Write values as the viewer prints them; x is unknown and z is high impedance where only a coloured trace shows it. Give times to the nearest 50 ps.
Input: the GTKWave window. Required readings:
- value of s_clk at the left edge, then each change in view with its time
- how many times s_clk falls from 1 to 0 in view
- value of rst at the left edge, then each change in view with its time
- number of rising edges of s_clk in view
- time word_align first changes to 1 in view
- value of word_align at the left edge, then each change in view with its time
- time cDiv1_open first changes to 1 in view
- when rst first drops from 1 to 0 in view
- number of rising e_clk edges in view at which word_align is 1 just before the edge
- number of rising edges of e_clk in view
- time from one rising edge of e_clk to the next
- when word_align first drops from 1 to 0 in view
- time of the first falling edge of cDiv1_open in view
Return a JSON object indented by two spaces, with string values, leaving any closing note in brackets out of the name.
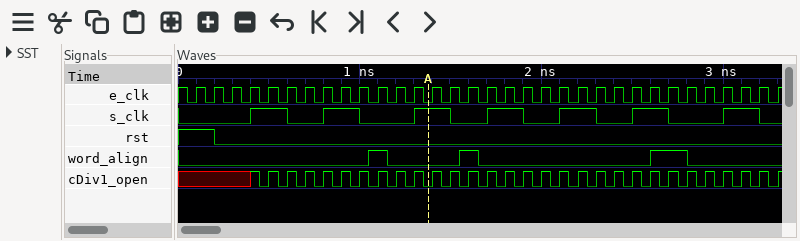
{
  "value of s_clk at the left edge, then each change in view with its time": "0, 1 at 400 ps, 0 at 600 ps, 1 at 800 ps, 0 at 1000 ps, 1 at 1300 ps, 0 at 1500 ps, 1 at 1700 ps, 0 at 1900 ps, 1 at 2100 ps, 0 at 2300 ps, 1 at 2500 ps, 0 at 2700 ps, 1 at 3000 ps, 0 at 3200 ps",
  "how many times s_clk falls from 1 to 0 in view": "7",
  "value of rst at the left edge, then each change in view with its time": "1, 0 at 200 ps",
  "number of rising edges of s_clk in view": "7",
  "time word_align first changes to 1 in view": "1050 ps",
  "value of word_align at the left edge, then each change in view with its time": "0, 1 at 1050 ps, 0 at 1150 ps, 1 at 1550 ps, 0 at 1650 ps, 1 at 2600 ps, 0 at 2800 ps",
  "time cDiv1_open first changes to 1 in view": "400 ps",
  "when rst first drops from 1 to 0 in view": "200 ps",
  "number of rising e_clk edges in view at which word_align is 1 just before the edge": "4",
  "number of rising edges of e_clk in view": "33",
  "time from one rising edge of e_clk to the next": "100 ps",
  "when word_align first drops from 1 to 0 in view": "1150 ps",
  "time of the first falling edge of cDiv1_open in view": "450 ps"
}
